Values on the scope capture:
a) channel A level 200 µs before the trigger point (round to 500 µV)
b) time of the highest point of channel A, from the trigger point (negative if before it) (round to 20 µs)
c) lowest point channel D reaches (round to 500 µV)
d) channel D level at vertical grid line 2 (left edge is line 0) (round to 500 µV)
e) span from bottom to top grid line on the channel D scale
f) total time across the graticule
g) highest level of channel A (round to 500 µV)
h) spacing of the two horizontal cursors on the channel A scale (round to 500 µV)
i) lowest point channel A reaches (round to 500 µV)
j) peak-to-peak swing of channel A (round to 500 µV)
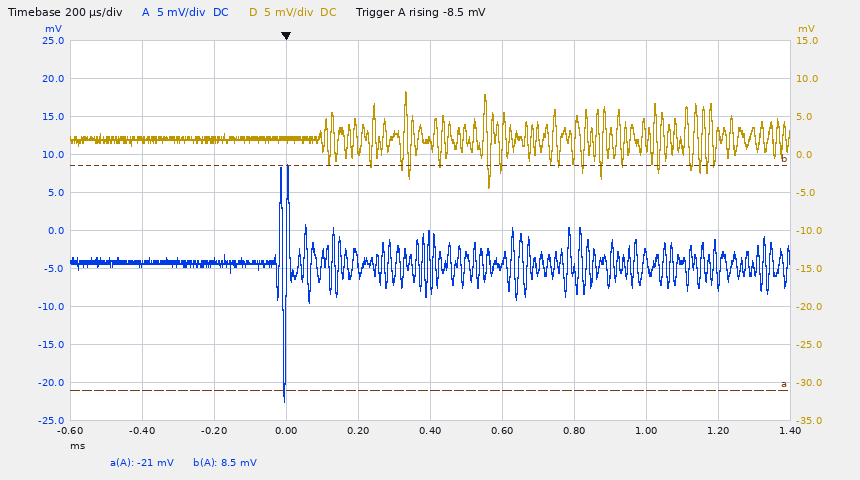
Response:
-4.0 mV
0 µs
-4.5 mV
2.0 mV
50 mV
2 ms
8.5 mV
29.5 mV
-22.5 mV
31.0 mV
